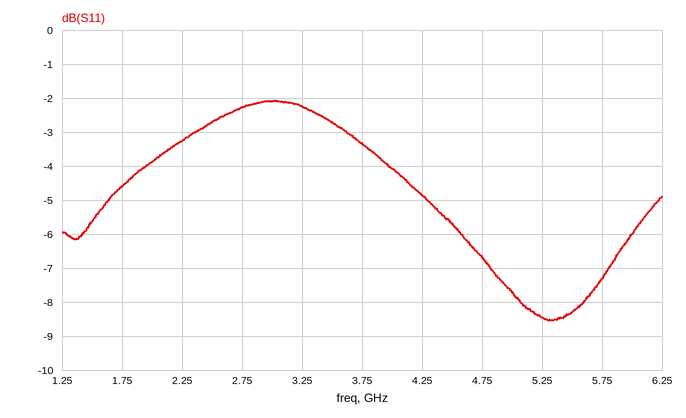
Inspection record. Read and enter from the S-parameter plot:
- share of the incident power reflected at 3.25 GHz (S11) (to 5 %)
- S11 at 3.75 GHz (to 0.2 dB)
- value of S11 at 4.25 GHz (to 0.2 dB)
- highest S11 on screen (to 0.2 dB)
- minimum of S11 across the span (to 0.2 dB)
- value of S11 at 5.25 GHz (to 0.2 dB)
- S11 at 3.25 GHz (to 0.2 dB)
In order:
60 %
-3.4 dB
-4.8 dB
-2.0 dB
-8.6 dB
-8.4 dB
-2.2 dB
